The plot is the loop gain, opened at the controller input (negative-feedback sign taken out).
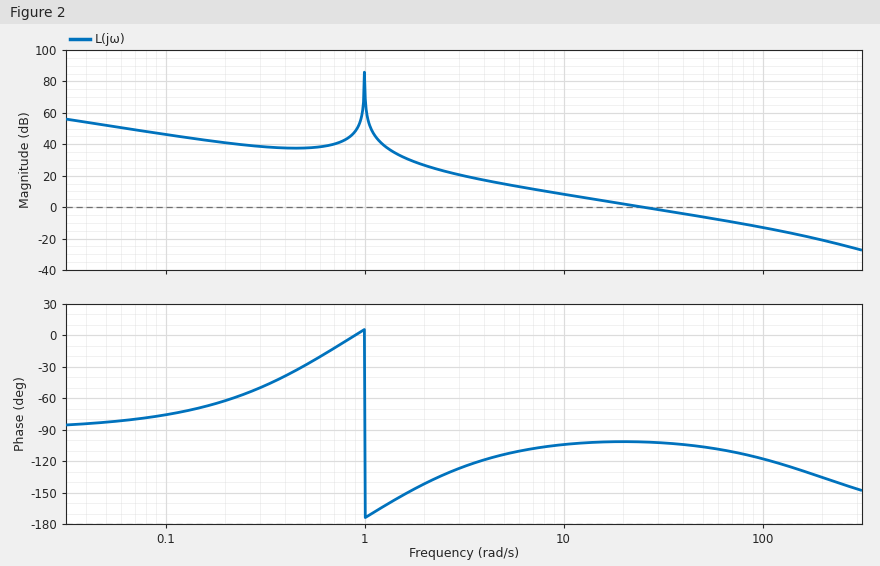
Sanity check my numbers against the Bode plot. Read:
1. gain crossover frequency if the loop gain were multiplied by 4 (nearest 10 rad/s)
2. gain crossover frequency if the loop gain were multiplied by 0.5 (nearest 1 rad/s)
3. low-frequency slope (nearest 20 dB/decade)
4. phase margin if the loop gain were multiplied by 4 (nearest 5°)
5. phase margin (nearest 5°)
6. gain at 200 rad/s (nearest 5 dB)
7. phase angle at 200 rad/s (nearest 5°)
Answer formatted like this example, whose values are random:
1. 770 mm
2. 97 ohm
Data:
1. 90 rad/s
2. 13 rad/s
3. -20 dB/decade
4. 65°
5. 80°
6. -20 dB
7. -135°
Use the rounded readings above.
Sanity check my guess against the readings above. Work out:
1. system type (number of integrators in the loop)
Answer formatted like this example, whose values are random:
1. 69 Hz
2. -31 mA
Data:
1. 1
